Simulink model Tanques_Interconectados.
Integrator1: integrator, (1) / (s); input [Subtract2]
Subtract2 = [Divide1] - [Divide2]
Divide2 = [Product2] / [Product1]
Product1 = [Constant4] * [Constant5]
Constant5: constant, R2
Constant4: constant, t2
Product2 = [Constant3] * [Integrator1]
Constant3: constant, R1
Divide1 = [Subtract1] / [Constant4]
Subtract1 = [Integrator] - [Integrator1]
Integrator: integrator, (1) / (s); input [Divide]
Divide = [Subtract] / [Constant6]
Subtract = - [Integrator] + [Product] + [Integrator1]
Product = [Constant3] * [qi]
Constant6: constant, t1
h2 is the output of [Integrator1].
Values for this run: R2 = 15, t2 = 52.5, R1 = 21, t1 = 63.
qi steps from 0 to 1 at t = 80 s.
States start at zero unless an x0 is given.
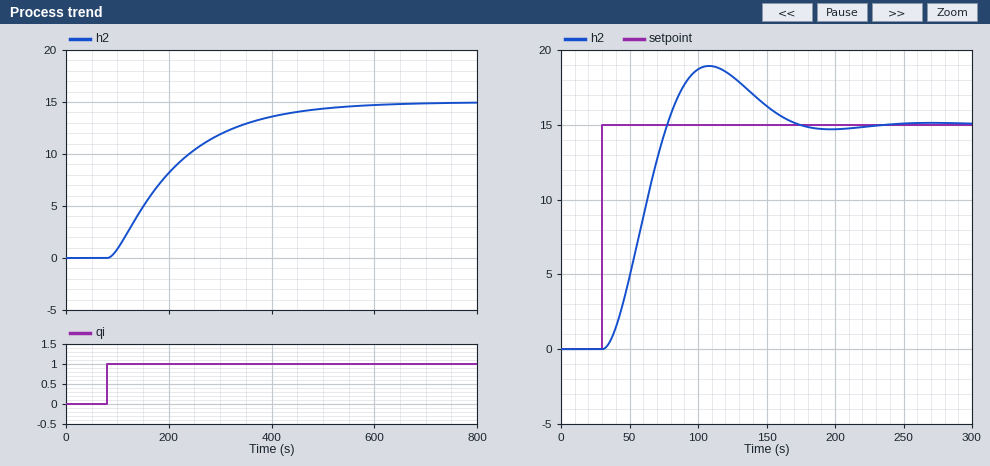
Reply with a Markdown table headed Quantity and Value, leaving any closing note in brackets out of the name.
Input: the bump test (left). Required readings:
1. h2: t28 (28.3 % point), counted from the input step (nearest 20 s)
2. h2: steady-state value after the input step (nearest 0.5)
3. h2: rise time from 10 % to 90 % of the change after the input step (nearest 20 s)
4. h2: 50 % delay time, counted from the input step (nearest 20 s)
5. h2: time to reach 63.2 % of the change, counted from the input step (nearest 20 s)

| Quantity | Value |
|---|---|
| h2: t28 (28.3 % point), counted from the input step | 60 s |
| h2: steady-state value after the input step | 15.0 |
| h2: rise time from 10 % to 90 % of the change after the input step | 280 s |
| h2: 50 % delay time, counted from the input step | 100 s |
| h2: time to reach 63.2 % of the change, counted from the input step | 140 s |
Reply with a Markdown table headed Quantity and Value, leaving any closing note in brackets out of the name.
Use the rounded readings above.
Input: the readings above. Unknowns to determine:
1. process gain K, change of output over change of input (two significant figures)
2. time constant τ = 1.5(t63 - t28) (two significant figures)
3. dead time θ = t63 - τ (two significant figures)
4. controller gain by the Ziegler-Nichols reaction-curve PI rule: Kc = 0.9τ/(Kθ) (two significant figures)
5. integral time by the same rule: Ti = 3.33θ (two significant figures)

| Quantity | Value |
|---|---|
| process gain K, change of output over change of input | 15 |
| time constant τ = 1.5(t63 - t28) | 120 s |
| dead time θ = t63 - τ | 20 s |
| controller gain by the Ziegler-Nichols reaction-curve PI rule: Kc = 0.9τ/(Kθ) | 0.36 |
| integral time by the same rule: Ti = 3.33θ | 67 s |
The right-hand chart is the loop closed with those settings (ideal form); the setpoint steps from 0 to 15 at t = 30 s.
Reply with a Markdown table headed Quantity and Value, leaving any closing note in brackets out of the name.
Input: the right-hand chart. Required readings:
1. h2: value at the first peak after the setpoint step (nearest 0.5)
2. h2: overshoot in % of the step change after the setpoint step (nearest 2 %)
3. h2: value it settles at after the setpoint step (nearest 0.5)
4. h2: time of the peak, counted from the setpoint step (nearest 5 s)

| Quantity | Value |
|---|---|
| h2: value at the first peak after the setpoint step | 19.0 |
| h2: overshoot in % of the step change after the setpoint step | 26 % |
| h2: value it settles at after the setpoint step | 15.0 |
| h2: time of the peak, counted from the setpoint step | 80 s |
